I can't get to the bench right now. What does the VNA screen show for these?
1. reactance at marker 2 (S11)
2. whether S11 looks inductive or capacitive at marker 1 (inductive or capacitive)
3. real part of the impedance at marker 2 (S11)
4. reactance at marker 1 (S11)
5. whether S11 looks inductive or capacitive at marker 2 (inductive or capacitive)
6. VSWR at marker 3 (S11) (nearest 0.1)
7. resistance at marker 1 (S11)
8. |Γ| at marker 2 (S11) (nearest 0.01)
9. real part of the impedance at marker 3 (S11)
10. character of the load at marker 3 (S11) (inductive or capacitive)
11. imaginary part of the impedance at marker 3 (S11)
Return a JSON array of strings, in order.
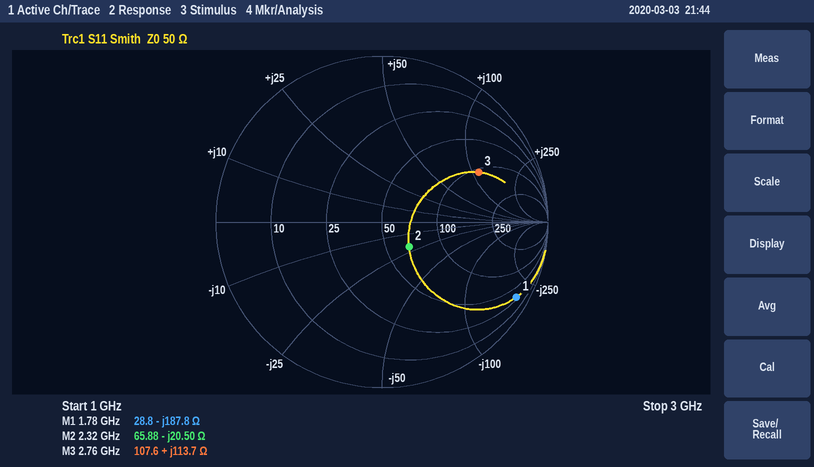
["-20.50 Ω", "capacitive", "65.88 Ω", "-187.8 Ω", "capacitive", "4.8", "28.8 Ω", "0.22", "107.6 Ω", "inductive", "+113.7 Ω"]
